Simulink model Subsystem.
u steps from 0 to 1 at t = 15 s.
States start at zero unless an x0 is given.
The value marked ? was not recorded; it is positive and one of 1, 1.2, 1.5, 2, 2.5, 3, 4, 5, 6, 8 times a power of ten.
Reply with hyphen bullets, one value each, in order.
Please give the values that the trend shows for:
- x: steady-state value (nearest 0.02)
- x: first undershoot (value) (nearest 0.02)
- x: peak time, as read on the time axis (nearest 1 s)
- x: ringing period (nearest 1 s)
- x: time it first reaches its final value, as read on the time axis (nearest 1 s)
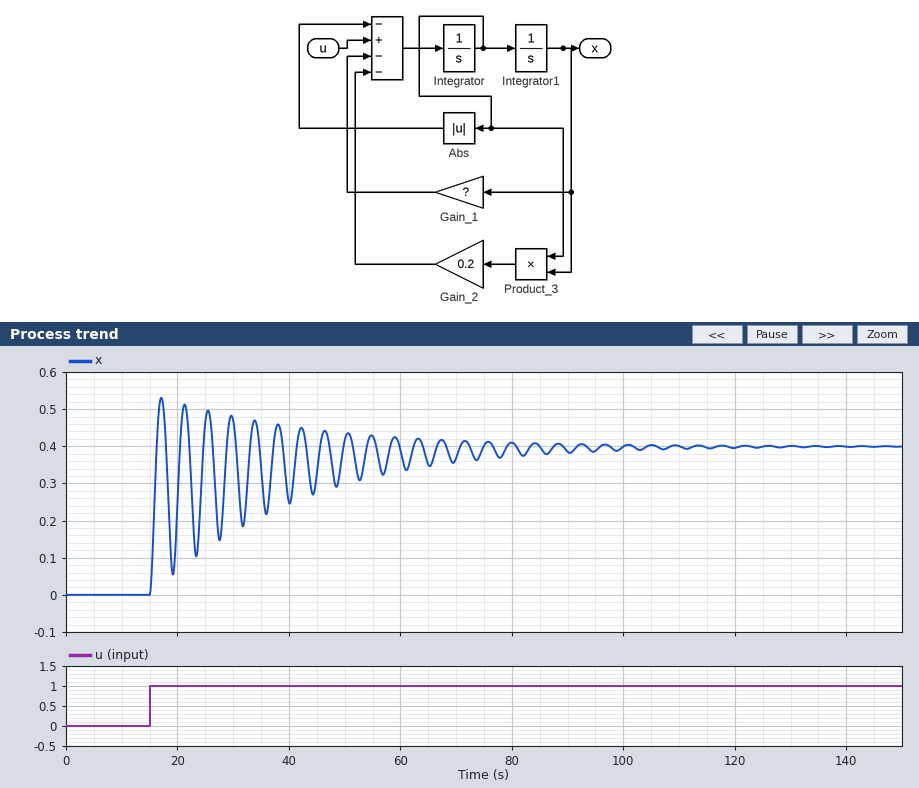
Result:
- 0.40
- 0.06
- 17 s
- 4 s
- 16 s
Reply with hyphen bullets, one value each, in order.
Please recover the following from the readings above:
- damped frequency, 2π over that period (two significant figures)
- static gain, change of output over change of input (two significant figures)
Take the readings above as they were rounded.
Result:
- 1.6 rad/s
- 0.40
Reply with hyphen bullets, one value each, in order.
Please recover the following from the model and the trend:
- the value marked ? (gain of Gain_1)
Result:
- 2.5
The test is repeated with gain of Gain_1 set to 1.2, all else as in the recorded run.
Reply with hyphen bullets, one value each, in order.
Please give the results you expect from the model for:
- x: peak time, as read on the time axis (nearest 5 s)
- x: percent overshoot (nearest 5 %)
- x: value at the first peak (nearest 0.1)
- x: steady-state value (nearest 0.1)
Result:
- 20 s
- 15 %
- 1.0
- 0.8
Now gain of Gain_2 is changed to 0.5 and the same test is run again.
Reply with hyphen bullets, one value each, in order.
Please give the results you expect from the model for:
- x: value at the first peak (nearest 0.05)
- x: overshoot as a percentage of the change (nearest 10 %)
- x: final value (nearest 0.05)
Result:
- 0.50
- 30 %
- 0.40
